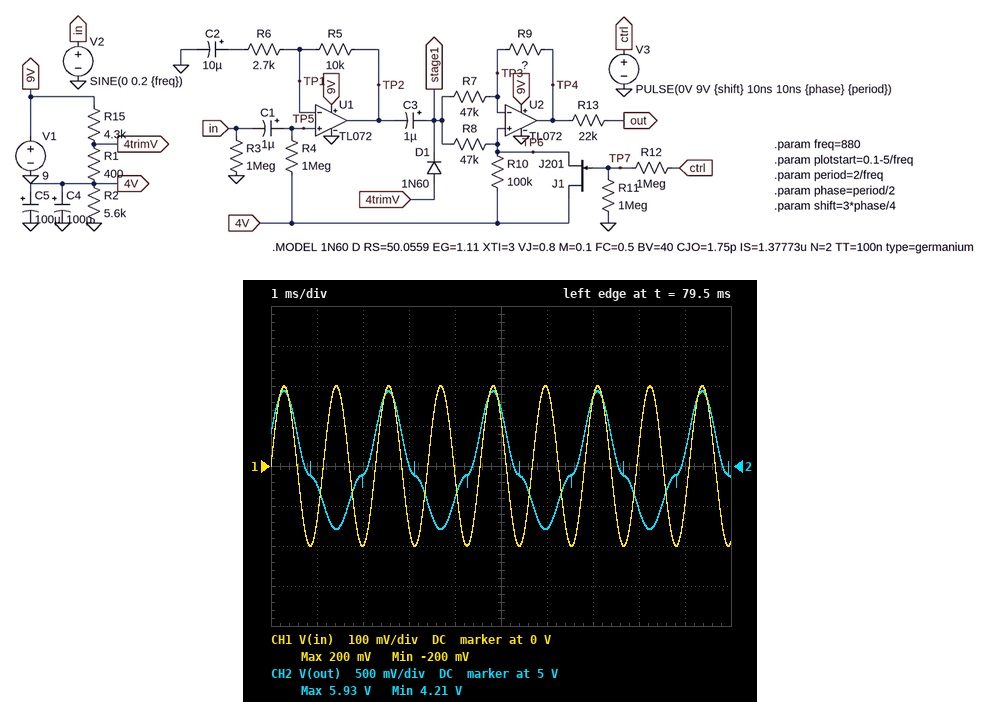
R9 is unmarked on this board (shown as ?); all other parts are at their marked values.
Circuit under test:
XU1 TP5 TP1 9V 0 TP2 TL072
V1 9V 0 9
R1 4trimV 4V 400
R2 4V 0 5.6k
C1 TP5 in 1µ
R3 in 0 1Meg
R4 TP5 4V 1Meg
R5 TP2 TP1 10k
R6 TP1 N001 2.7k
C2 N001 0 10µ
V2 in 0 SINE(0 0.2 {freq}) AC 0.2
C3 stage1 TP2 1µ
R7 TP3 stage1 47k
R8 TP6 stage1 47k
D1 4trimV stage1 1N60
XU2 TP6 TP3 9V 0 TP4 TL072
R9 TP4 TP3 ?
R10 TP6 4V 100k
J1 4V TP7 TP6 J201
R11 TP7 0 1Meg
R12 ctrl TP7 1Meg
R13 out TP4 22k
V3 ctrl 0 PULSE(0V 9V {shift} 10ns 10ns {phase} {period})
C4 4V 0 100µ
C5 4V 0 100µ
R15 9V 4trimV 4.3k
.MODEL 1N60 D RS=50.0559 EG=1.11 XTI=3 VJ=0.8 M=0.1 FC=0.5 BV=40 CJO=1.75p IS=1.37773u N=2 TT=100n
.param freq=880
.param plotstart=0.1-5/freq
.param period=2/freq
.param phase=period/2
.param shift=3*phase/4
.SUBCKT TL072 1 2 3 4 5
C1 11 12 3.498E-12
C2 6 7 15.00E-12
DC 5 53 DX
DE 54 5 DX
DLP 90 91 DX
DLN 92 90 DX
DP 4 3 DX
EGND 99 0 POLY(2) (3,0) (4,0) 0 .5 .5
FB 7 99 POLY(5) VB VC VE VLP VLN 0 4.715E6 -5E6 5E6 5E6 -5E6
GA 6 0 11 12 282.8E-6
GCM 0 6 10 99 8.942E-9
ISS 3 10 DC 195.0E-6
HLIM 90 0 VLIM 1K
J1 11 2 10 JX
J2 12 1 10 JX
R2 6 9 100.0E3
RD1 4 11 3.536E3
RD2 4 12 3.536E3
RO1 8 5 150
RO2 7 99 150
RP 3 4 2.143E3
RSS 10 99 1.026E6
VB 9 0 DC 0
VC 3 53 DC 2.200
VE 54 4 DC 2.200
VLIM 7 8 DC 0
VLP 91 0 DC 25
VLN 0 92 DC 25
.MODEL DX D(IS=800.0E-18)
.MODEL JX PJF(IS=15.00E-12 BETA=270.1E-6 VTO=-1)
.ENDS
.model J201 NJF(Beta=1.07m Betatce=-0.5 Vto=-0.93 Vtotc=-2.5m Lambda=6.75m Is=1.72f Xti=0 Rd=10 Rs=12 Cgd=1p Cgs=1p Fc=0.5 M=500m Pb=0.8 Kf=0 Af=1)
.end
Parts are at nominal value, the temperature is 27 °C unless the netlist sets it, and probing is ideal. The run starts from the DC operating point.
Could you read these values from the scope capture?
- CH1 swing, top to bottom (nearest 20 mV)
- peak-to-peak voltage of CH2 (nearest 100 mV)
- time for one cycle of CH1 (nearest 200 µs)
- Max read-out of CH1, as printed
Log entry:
400 mV
1.7 V
1.2 ms
200 mV
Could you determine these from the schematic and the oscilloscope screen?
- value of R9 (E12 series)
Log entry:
18 kΩ
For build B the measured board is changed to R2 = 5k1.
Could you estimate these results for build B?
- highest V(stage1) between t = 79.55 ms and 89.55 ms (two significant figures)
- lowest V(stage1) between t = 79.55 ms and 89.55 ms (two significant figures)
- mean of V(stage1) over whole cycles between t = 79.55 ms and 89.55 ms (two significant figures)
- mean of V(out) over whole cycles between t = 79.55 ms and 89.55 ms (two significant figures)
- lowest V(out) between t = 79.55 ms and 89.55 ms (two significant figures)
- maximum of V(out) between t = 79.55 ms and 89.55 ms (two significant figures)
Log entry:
6.6 V
4.7 V
5.6 V
4.8 V
4.0 V
5.7 V
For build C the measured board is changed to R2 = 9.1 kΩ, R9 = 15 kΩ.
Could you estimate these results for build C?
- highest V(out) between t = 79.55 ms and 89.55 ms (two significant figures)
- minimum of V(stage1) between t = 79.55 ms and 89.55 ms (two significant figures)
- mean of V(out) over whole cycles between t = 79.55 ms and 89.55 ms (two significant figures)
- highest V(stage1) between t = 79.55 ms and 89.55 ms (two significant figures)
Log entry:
7.0 V
5.9 V
6.5 V
7.8 V
